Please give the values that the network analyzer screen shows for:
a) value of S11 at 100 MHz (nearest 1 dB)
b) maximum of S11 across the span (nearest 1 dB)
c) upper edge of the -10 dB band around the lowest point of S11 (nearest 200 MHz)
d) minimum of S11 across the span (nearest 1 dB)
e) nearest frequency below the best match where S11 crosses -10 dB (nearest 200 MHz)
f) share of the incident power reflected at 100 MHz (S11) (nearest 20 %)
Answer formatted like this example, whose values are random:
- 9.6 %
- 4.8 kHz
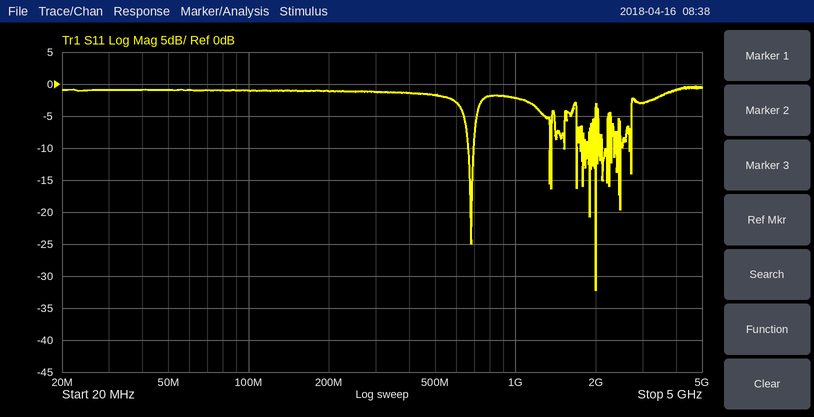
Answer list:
- -1 dB
- 0 dB
- 2.0 GHz
- -32 dB
- 2.0 GHz
- 80 %
